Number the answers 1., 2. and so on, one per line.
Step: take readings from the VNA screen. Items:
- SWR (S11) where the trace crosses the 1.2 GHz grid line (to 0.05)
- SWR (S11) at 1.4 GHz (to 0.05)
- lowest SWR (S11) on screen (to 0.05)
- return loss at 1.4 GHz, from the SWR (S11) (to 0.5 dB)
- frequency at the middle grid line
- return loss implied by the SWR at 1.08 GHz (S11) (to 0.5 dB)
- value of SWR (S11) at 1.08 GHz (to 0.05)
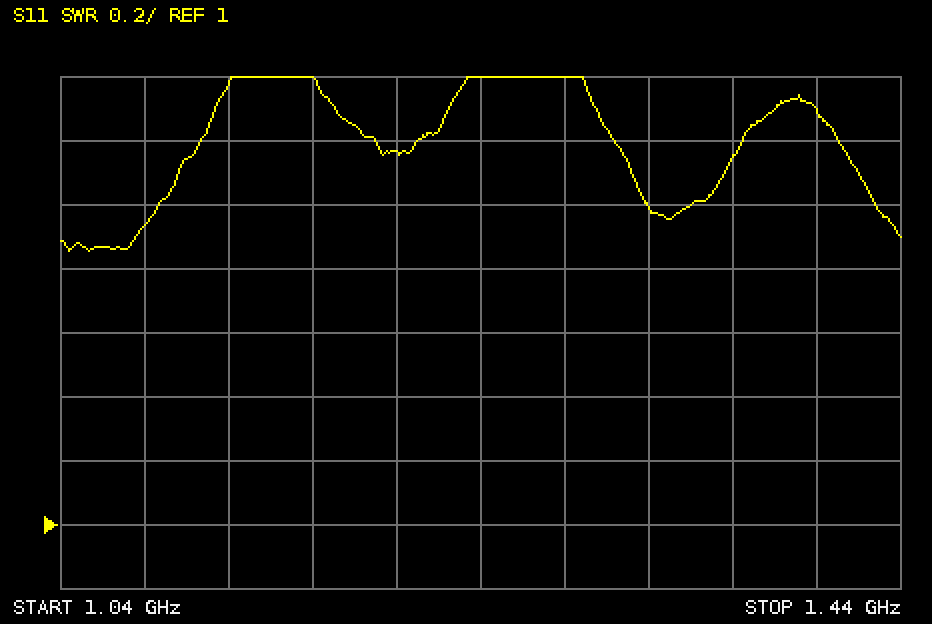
1. 2.15
2. 2.30
3. 1.85
4. 8.0 dB
5. 1.24 GHz
6. 10.0 dB
7. 1.95
